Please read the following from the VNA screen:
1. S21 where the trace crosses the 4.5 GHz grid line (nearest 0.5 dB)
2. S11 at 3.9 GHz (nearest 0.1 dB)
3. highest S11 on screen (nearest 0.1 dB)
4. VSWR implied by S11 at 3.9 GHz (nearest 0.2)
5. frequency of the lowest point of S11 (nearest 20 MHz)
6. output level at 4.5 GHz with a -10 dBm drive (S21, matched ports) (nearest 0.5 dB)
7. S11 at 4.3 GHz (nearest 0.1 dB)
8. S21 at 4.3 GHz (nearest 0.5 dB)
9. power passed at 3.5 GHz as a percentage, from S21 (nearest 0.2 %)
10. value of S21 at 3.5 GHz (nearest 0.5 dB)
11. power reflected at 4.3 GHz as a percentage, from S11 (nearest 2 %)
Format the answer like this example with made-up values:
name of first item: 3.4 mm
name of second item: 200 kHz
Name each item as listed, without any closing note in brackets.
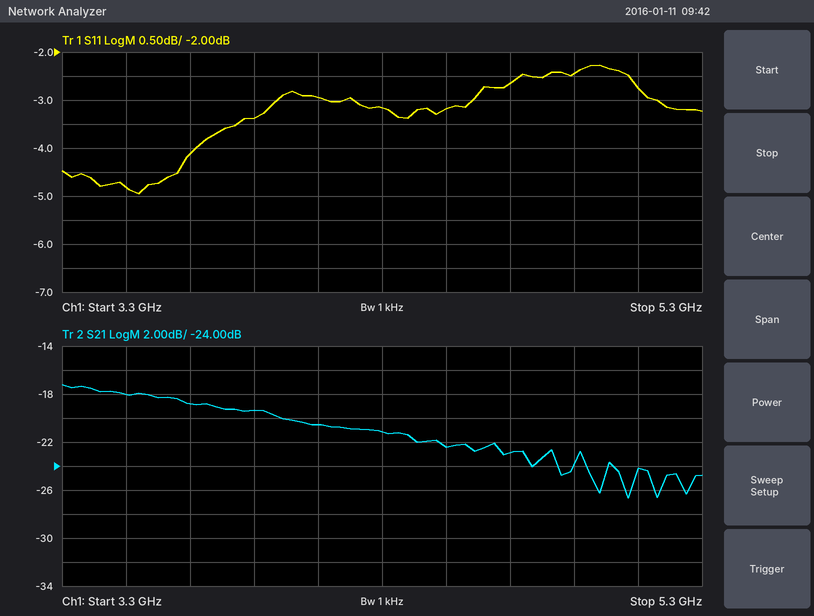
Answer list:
S21 where the trace crosses the 4.5 GHz grid line: -22.5 dB
S11 at 3.9 GHz: -3.4 dB
highest S11 on screen: -2.3 dB
VSWR implied by S11 at 3.9 GHz: 5.2
frequency of the lowest point of S11: 3.54 GHz
output level at 4.5 GHz with a -10 dBm drive (S21, matched ports): -32.5 dBm
S11 at 4.3 GHz: -3.2 dB
S21 at 4.3 GHz: -21.0 dB
power passed at 3.5 GHz as a percentage, from S21: 1.6 %
value of S21 at 3.5 GHz: -18.0 dB
power reflected at 4.3 GHz as a percentage, from S11: 48 %
